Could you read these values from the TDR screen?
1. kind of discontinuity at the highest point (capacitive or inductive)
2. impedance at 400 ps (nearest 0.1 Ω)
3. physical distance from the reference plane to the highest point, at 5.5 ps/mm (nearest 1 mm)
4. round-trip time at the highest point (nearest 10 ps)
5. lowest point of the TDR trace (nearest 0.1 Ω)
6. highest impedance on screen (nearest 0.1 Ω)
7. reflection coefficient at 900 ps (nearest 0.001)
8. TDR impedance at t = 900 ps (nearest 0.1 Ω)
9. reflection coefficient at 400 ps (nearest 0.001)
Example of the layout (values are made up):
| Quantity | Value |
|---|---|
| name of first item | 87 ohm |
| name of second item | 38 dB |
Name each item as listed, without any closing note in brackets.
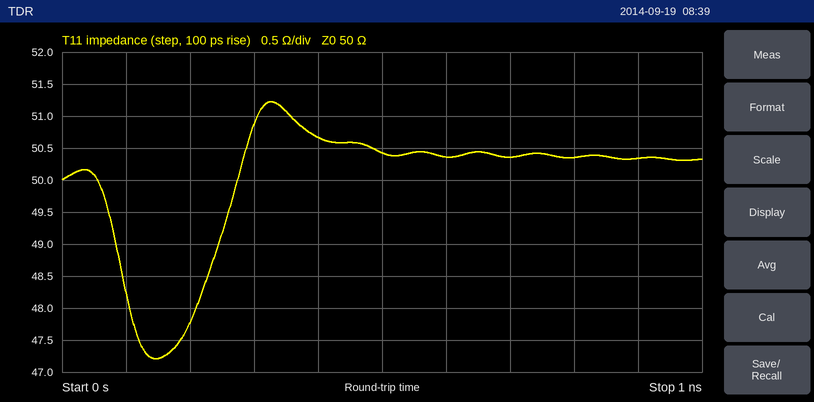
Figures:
| Quantity | Value |
|---|---|
| kind of discontinuity at the highest point | inductive |
| impedance at 400 ps | 50.7 Ω |
| physical distance from the reference plane to the highest point, at 5.5 ps/mm | 30 mm |
| round-trip time at the highest point | 330 ps |
| lowest point of the TDR trace | 47.2 Ω |
| highest impedance on screen | 51.2 Ω |
| reflection coefficient at 900 ps | +0.003 |
| TDR impedance at t = 900 ps | 50.3 Ω |
| reflection coefficient at 400 ps | +0.007 |
